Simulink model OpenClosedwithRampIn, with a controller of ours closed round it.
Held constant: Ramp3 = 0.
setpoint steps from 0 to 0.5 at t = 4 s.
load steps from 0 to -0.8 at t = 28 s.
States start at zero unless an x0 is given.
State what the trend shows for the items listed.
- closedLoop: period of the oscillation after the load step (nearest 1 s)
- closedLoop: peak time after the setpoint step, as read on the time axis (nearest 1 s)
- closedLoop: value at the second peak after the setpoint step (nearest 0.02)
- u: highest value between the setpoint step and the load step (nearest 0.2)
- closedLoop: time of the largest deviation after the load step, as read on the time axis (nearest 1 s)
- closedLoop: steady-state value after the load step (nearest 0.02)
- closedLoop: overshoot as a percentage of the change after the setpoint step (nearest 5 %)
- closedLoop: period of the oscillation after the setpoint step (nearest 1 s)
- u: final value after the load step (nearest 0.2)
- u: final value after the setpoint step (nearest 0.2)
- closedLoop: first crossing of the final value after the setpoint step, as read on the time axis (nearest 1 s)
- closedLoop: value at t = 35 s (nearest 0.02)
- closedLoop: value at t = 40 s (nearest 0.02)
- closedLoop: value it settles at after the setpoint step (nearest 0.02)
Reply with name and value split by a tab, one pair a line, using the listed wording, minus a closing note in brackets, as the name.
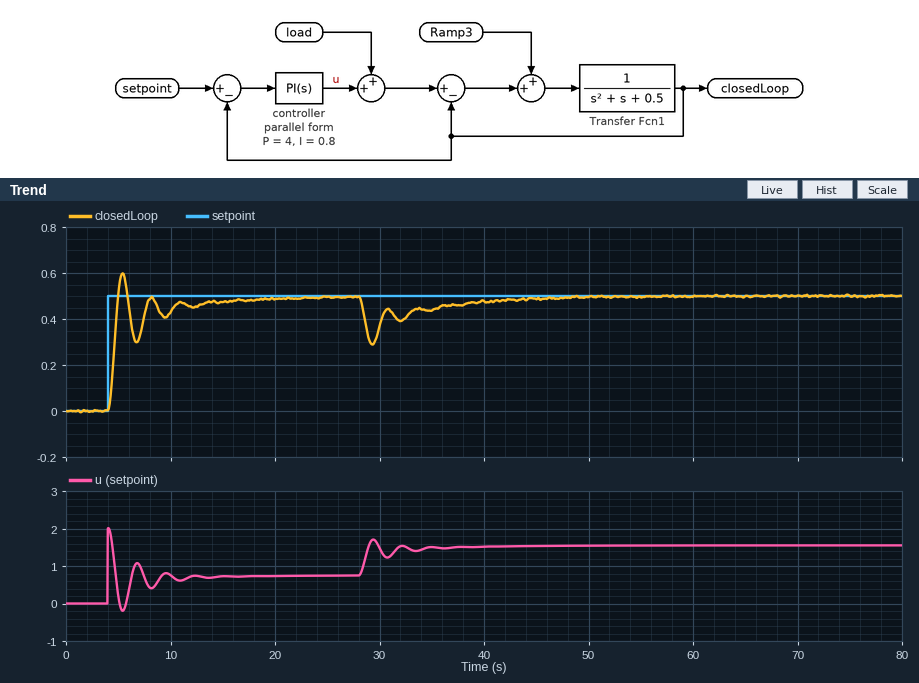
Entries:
closedLoop: period of the oscillation after the load step	3 s
closedLoop: peak time after the setpoint step, as read on the time axis	5 s
closedLoop: value at the second peak after the setpoint step	0.50
u: highest value between the setpoint step and the load step	2.0
closedLoop: time of the largest deviation after the load step, as read on the time axis	29 s
closedLoop: steady-state value after the load step	0.50
closedLoop: overshoot as a percentage of the change after the setpoint step	20 %
closedLoop: period of the oscillation after the setpoint step	3 s
u: final value after the load step	1.6
u: final value after the setpoint step	0.8
closedLoop: first crossing of the final value after the setpoint step, as read on the time axis	5 s
closedLoop: value at t = 35 s	0.44
closedLoop: value at t = 40 s	0.48
closedLoop: value it settles at after the setpoint step	0.50
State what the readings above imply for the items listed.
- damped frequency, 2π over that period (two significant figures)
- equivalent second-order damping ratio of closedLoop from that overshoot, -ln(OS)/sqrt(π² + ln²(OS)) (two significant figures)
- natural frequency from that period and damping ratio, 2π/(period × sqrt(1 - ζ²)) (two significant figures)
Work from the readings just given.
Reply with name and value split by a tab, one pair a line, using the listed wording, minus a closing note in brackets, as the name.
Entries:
damped frequency, 2π over that period	2.1 rad/s
equivalent second-order damping ratio of closedLoop from that overshoot, -ln(OS)/sqrt(π² + ln²(OS))	0.46
natural frequency from that period and damping ratio, 2π/(period × sqrt(1 - ζ²))	2.4 rad/s
